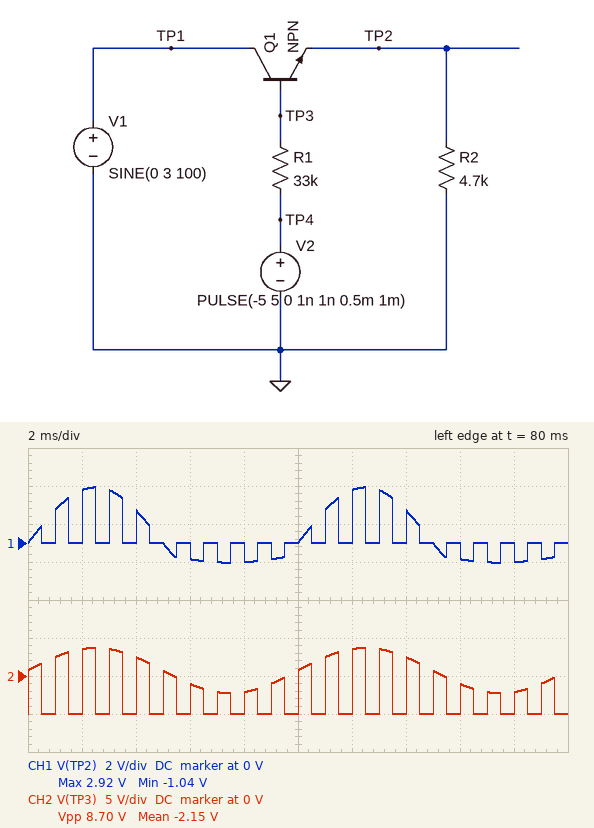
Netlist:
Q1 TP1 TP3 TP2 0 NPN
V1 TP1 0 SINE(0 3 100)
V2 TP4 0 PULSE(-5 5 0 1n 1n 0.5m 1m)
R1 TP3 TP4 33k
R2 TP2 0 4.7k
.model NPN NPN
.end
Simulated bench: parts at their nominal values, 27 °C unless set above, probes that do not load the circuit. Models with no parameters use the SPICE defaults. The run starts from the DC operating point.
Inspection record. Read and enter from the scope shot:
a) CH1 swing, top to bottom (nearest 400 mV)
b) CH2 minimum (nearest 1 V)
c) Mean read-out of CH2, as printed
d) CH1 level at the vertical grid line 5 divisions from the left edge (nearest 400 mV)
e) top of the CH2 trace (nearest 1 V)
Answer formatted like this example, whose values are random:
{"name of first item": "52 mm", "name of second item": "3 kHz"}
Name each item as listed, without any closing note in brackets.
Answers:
{"CH1 swing, top to bottom": "4.0 V", "CH2 minimum": "-5 V", "Mean read-out of CH2, as printed": "-2.15 V", "CH1 level at the vertical grid line 5 divisions from the left edge": "0 V", "top of the CH2 trace": "4 V"}
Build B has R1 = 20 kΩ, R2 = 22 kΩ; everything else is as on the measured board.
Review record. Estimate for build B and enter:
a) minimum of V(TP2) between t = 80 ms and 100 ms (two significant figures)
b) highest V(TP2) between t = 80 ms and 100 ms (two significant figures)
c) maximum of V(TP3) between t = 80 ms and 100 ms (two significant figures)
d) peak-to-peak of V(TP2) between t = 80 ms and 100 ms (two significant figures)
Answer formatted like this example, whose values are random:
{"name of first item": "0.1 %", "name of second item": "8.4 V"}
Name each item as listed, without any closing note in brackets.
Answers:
{"minimum of V(TP2) between t = 80 ms and 100 ms": "-3.0 V", "highest V(TP2) between t = 80 ms and 100 ms": "3.0 V", "maximum of V(TP3) between t = 80 ms and 100 ms": "3.7 V", "peak-to-peak of V(TP2) between t = 80 ms and 100 ms": "6.0 V"}
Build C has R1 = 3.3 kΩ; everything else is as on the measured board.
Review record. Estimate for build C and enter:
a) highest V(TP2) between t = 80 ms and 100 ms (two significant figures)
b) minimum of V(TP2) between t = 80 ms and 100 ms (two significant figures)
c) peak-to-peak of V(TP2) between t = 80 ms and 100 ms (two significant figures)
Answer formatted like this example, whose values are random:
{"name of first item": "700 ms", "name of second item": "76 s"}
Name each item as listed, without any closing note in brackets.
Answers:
{"highest V(TP2) between t = 80 ms and 100 ms": "3.0 V", "minimum of V(TP2) between t = 80 ms and 100 ms": "-3.0 V", "peak-to-peak of V(TP2) between t = 80 ms and 100 ms": "6.0 V"}
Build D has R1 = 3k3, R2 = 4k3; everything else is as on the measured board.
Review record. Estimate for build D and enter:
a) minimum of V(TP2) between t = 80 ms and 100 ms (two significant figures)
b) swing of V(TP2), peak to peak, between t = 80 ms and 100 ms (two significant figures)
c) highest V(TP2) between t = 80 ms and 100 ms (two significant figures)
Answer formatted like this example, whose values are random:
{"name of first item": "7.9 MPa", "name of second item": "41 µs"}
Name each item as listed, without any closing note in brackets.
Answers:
{"minimum of V(TP2) between t = 80 ms and 100 ms": "-3.0 V", "swing of V(TP2), peak to peak, between t = 80 ms and 100 ms": "6.0 V", "highest V(TP2) between t = 80 ms and 100 ms": "3.0 V"}
